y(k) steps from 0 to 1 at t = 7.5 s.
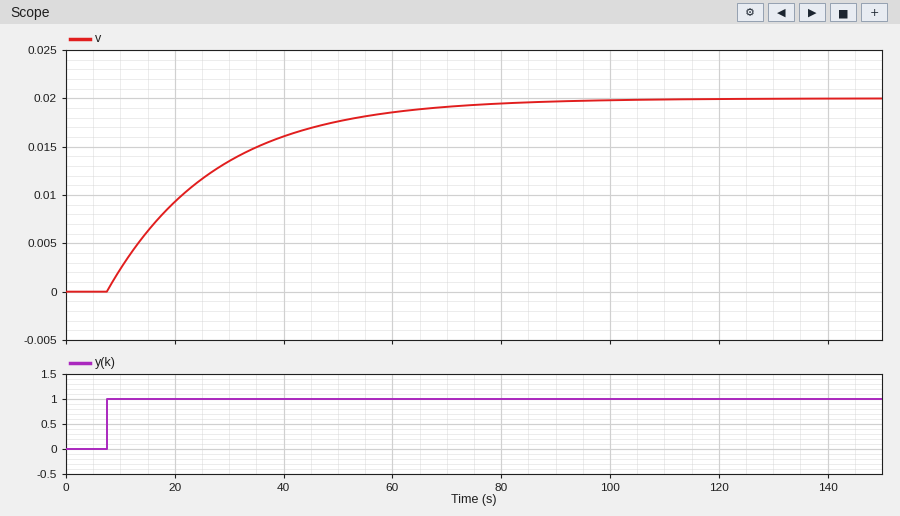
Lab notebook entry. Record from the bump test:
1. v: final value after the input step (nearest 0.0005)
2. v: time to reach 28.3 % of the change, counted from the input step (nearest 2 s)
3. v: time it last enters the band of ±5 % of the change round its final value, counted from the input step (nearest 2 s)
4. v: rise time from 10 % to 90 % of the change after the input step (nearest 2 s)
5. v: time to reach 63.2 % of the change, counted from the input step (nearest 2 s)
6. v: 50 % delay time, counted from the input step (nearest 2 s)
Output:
0.0200
6 s
60 s
44 s
20 s
14 s
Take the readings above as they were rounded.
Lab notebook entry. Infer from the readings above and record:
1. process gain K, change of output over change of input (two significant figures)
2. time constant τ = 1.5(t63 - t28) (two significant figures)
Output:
0.020
21 s
